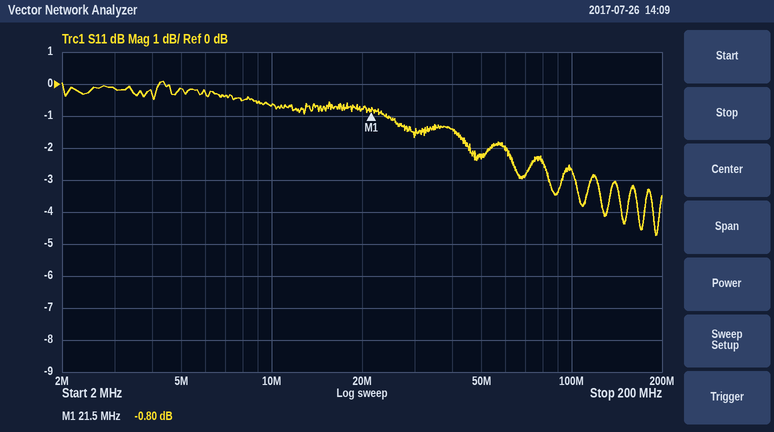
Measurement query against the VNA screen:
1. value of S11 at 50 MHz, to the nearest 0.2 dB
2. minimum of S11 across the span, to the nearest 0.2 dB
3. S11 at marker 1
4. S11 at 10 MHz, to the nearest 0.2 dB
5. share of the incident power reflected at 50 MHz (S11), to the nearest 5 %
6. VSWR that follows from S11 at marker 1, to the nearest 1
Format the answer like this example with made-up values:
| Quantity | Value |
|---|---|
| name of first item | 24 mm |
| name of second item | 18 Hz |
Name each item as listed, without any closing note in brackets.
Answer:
| Quantity | Value |
|---|---|
| value of S11 at 50 MHz, to the nearest 0.2 dB | -2.2 dB |
| minimum of S11 across the span, to the nearest 0.2 dB | -4.8 dB |
| S11 at marker 1 | -0.80 dB |
| S11 at 10 MHz, to the nearest 0.2 dB | -0.6 dB |
| share of the incident power reflected at 50 MHz (S11), to the nearest 5 % | 60 % |
| VSWR that follows from S11 at marker 1, to the nearest 1 | 22 |
